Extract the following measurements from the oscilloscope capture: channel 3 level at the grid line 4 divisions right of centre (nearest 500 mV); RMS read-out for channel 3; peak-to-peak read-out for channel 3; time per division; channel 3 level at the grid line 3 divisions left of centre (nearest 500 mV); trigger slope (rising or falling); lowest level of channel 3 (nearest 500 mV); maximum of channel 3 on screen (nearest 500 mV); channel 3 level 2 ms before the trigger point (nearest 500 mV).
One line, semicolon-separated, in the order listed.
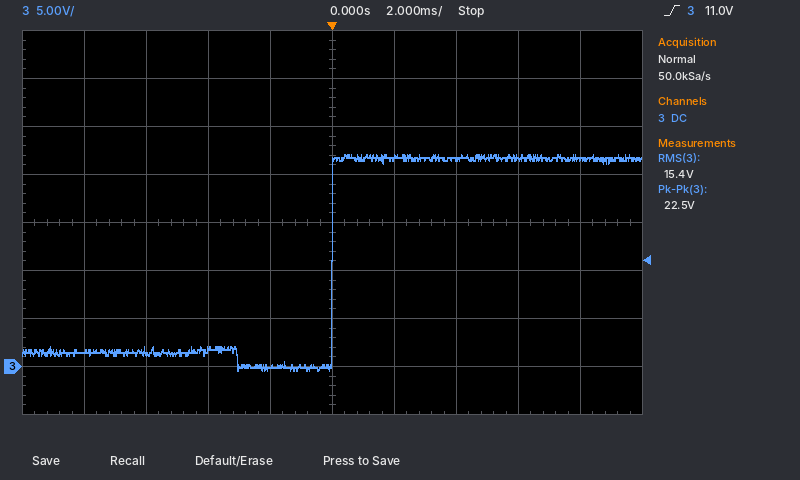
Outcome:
21.5 V; 15.4 V; 22.5 V; 2 ms; 1.5 V; rising; -500 mV; 22.0 V; 0.0 V
